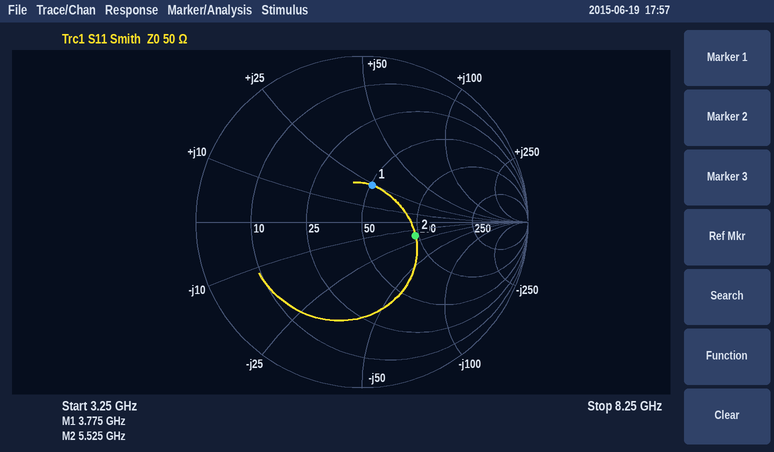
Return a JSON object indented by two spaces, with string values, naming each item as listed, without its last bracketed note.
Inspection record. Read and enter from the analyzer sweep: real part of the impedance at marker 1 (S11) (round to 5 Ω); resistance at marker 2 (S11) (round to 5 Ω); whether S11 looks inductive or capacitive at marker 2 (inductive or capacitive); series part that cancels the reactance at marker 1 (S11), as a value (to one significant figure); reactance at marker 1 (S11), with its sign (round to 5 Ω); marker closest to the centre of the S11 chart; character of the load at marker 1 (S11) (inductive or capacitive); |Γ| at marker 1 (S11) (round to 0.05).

{
  "real part of the impedance at marker 1 (S11)": "50 Ω",
  "resistance at marker 2 (S11)": "95 Ω",
  "whether S11 looks inductive or capacitive at marker 2": "capacitive",
  "series part that cancels the reactance at marker 1 (S11), as a value": "2 pF",
  "reactance at marker 1 (S11), with its sign": "+25 Ω",
  "marker closest to the centre of the S11 chart": "marker 1",
  "character of the load at marker 1 (S11)": "inductive",
  "|Γ| at marker 1 (S11)": "0.25"
}
